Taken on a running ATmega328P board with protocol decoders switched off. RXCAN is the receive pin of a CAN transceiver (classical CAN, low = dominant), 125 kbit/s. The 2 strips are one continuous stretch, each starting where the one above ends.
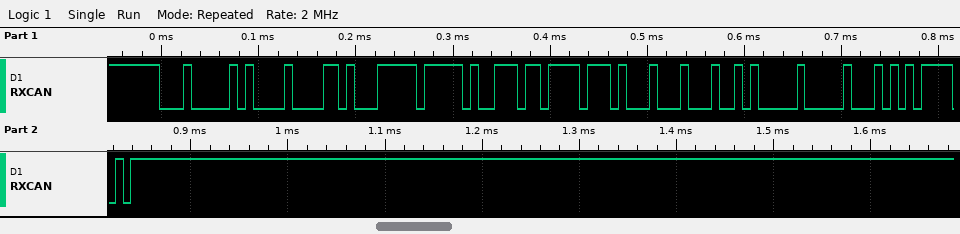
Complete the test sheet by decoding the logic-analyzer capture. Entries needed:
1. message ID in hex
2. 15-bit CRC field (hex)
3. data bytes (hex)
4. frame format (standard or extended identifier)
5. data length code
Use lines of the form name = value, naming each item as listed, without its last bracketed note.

message ID in hex = 0x102
15-bit CRC field = 0x055E
data bytes = 68 FF E7 6F 74 44 4A 00
frame format = standard
data length code = 8
